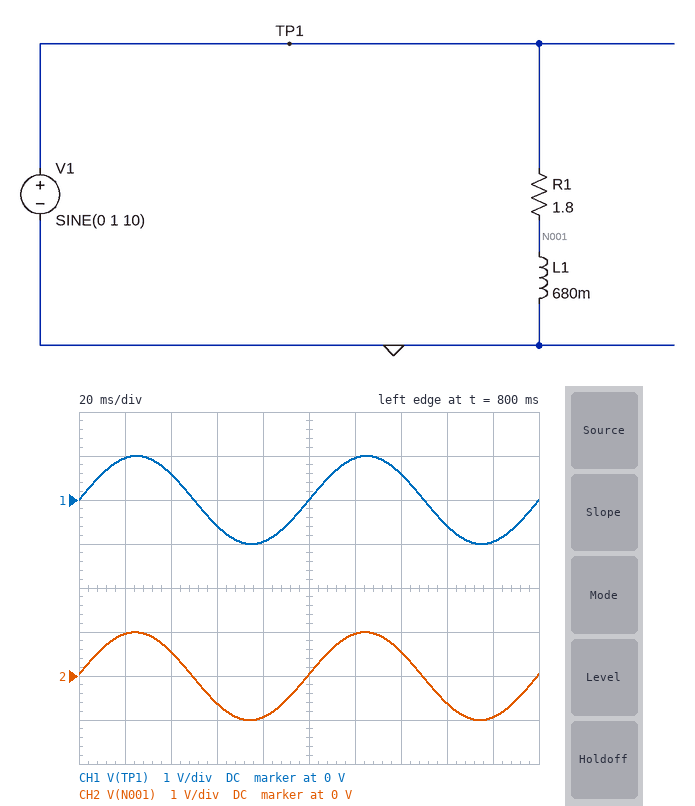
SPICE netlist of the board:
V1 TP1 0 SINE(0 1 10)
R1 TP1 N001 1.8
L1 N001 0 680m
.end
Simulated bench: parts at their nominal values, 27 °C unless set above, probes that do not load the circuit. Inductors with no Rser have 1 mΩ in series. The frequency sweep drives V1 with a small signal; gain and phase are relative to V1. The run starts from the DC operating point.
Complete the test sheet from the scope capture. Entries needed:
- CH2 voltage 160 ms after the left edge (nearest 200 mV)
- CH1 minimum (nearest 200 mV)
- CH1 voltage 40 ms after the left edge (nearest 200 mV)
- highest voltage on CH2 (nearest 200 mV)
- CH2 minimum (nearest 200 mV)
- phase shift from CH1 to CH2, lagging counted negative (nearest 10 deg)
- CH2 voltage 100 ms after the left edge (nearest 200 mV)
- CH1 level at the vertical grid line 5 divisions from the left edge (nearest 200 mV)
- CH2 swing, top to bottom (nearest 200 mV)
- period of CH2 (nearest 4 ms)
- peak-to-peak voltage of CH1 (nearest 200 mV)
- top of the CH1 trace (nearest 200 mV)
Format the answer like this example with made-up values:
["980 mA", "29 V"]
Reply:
["-600 mV", "-1.0 V", "600 mV", "1.0 V", "-1.0 V", "0 deg", "0 V", "0 V", "2.0 V", "100 ms", "2.0 V", "1.0 V"]
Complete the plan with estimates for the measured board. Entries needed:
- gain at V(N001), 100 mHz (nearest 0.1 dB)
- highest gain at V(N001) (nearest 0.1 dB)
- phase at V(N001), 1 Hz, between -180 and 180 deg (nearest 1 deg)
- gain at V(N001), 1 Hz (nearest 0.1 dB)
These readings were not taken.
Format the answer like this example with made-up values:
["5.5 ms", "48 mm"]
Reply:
["-12.7 dB", "0 dB", "23 deg", "-0.7 dB"]
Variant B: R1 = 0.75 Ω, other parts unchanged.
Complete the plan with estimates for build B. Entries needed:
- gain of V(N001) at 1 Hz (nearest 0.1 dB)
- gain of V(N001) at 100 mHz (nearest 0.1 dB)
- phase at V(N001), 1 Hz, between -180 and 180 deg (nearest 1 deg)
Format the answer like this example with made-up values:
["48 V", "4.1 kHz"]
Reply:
["-0.1 dB", "-6.1 dB", "10 deg"]
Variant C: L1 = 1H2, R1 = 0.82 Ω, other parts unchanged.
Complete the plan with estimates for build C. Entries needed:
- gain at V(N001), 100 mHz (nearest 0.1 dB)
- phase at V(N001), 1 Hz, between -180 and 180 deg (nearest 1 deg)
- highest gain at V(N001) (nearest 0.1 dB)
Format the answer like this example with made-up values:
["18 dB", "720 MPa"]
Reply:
["-3.4 dB", "6 deg", "0 dB"]
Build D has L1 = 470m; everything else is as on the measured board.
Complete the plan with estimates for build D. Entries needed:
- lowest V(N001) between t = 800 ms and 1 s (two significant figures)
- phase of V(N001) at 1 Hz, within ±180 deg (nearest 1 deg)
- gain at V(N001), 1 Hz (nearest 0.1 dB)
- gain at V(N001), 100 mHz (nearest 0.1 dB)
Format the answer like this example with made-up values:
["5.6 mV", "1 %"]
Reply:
["-1.0 V", "31 deg", "-1.4 dB", "-15.8 dB"]
